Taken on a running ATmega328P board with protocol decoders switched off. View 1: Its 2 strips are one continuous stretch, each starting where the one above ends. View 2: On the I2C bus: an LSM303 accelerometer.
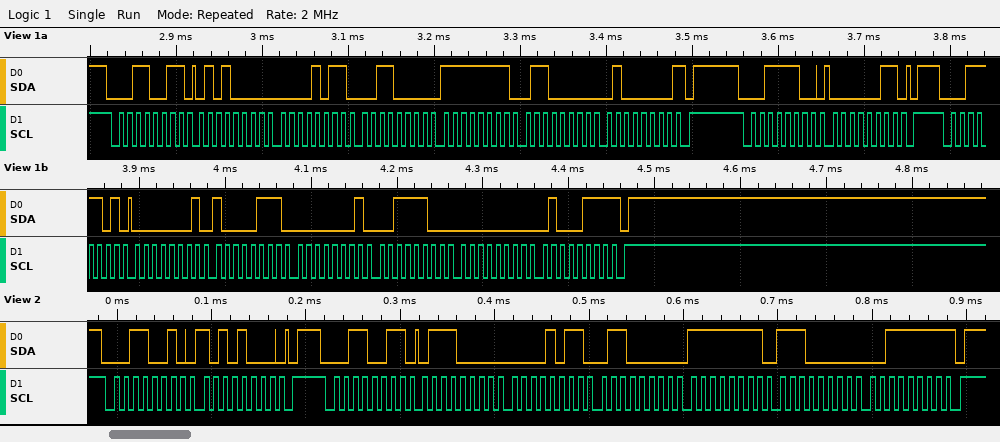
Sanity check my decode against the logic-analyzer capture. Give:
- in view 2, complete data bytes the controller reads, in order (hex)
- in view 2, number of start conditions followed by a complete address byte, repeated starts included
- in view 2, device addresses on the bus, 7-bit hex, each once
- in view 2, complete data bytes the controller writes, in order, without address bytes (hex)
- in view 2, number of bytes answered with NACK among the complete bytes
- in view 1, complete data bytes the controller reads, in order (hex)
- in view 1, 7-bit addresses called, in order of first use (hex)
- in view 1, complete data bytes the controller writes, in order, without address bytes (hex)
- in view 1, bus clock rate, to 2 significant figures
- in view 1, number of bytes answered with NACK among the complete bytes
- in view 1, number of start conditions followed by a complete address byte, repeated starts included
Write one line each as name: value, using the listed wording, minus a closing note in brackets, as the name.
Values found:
in view 2, complete data bytes the controller reads, in order: 70 0B 60 FF E0 3F
in view 2, number of start conditions followed by a complete address byte, repeated starts included: 2
in view 2, device addresses on the bus, 7-bit hex, each once: 0x19
in view 2, complete data bytes the controller writes, in order, without address bytes: A8
in view 2, number of bytes answered with NACK among the complete bytes: 1
in view 1, complete data bytes the controller reads, in order: 50 0B 30 FF 60 40 01 87 01 3C 00 47
in view 1, 7-bit addresses called, in order of first use: 0x19 0x1E
in view 1, complete data bytes the controller writes, in order, without address bytes: 03
in view 1, bus clock rate, to 2 significant figures: 100 kHz
in view 1, number of bytes answered with NACK among the complete bytes: 2
in view 1, number of start conditions followed by a complete address byte, repeated starts included: 3
